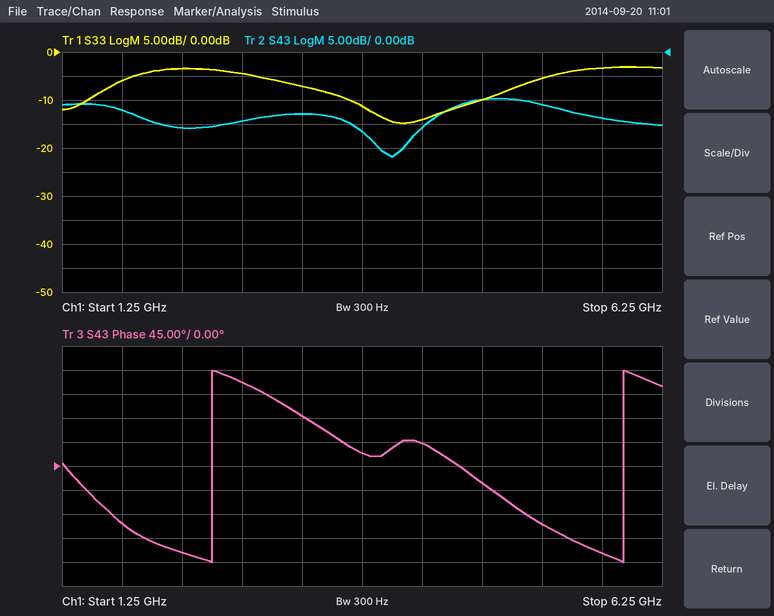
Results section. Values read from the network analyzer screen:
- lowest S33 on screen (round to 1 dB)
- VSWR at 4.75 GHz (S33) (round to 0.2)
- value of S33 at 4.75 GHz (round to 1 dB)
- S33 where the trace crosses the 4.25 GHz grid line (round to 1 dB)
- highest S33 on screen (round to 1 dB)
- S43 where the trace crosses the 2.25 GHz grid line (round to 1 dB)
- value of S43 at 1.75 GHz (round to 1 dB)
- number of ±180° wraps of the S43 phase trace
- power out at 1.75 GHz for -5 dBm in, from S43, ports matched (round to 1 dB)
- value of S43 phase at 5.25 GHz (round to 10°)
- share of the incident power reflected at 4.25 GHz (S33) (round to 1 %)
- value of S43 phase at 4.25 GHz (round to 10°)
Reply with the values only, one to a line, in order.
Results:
-15 dB
2.0
-10 dB
-14 dB
-3 dB
-16 dB
-12 dB
2
-17 dBm
-110°
4 %
40°
